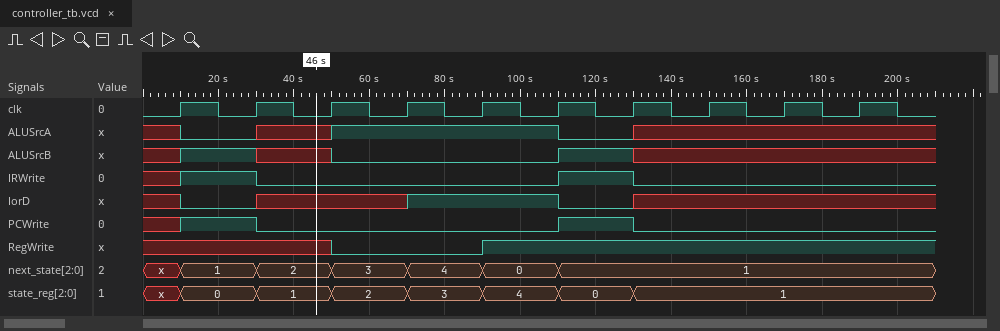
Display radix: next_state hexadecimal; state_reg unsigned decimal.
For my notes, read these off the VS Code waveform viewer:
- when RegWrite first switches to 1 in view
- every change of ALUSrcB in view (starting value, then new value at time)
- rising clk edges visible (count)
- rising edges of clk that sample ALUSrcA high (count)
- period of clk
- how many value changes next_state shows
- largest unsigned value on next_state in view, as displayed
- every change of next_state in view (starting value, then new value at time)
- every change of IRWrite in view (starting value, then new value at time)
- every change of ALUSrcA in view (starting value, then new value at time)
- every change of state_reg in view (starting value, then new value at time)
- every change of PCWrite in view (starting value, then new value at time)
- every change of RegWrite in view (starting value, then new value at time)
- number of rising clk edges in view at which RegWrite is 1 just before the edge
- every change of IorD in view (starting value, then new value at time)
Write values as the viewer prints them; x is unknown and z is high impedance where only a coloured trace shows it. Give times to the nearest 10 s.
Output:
90 s
x, 1 at 10 s, x at 30 s, 0 at 50 s, 1 at 110 s, x at 130 s
10
3
20 s
6
4
x, 1 at 10 s, 2 at 30 s, 3 at 50 s, 4 at 70 s, 0 at 90 s, 1 at 110 s
x, 1 at 10 s, 0 at 30 s, 1 at 110 s, 0 at 130 s
x, 0 at 10 s, x at 30 s, 1 at 50 s, 0 at 110 s, x at 130 s
x, 0 at 10 s, 1 at 30 s, 2 at 50 s, 3 at 70 s, 4 at 90 s, 0 at 110 s, 1 at 130 s
x, 1 at 10 s, 0 at 30 s, 1 at 110 s, 0 at 130 s
x, 0 at 50 s, 1 at 90 s
5
x, 0 at 10 s, x at 30 s, 1 at 70 s, 0 at 110 s, x at 130 s
